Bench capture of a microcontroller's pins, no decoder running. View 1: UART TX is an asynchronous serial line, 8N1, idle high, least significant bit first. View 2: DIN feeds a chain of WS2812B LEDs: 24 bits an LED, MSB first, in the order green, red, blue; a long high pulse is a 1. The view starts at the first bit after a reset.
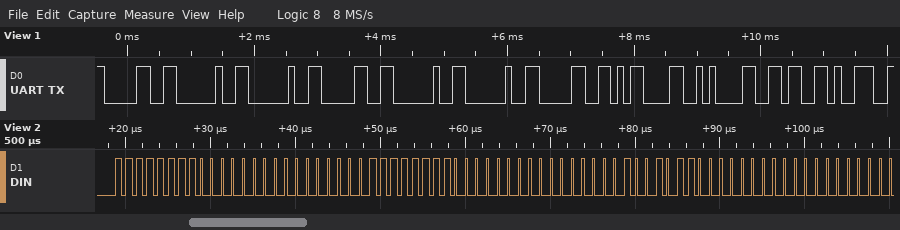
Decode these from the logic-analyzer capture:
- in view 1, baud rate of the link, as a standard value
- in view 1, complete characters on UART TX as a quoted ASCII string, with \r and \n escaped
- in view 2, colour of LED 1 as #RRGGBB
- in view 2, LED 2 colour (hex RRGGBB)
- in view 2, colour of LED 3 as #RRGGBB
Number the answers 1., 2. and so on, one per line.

1. 9600 baud
2. "0  0  0\r\n69"
3. #00FF00
4. #00FF00
5. #009600
